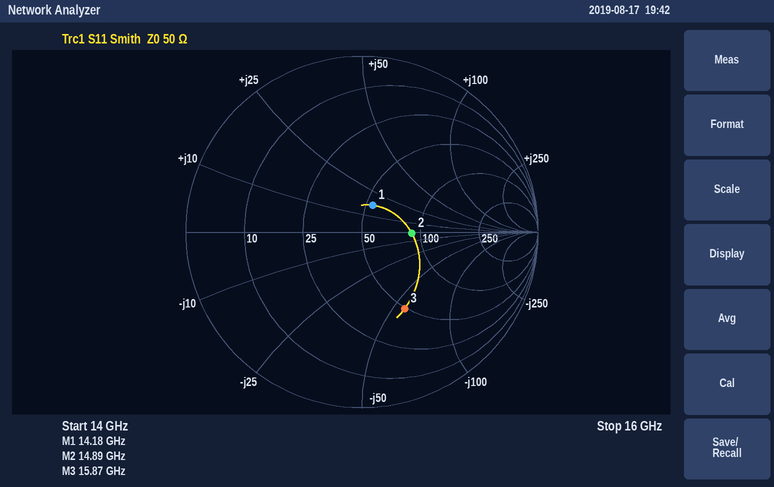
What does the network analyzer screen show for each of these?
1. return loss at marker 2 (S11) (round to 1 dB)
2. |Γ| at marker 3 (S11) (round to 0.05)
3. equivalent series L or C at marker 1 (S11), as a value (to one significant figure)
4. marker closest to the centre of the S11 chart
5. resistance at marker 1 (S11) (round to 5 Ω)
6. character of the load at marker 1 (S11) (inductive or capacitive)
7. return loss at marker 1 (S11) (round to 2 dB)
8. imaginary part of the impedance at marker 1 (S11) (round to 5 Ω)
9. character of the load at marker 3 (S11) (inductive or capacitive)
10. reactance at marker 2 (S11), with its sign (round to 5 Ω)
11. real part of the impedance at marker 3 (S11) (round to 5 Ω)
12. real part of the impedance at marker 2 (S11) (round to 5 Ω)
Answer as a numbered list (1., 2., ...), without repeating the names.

1. 11 dB
2. 0.50
3. 200 pH
4. marker 1
5. 55 Ω
6. inductive
7. 16 dB
8. +15 Ω
9. capacitive
10. 0 Ω
11. 50 Ω
12. 90 Ω
